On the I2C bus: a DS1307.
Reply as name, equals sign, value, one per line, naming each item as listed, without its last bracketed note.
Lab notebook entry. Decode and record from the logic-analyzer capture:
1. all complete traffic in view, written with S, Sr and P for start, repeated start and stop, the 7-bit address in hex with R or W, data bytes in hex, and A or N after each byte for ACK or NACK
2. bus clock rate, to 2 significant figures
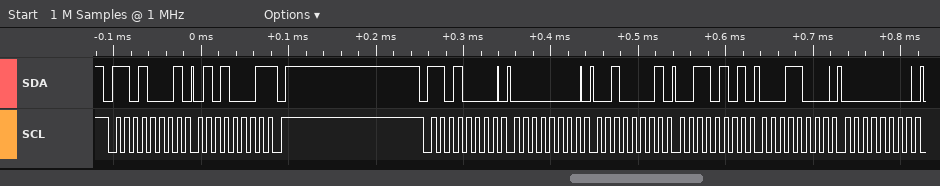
all complete traffic in view, written with S, Sr and P for start, repeated start and stop, the 7-bit address in hex with R or W, data bytes in hex, and A or N after each byte for ACK or NACK = S 68R A 51 N P S 68W A 00 A 21 A 35 A 18 A 00 A
bus clock rate, to 2 significant figures = 100 kHz
